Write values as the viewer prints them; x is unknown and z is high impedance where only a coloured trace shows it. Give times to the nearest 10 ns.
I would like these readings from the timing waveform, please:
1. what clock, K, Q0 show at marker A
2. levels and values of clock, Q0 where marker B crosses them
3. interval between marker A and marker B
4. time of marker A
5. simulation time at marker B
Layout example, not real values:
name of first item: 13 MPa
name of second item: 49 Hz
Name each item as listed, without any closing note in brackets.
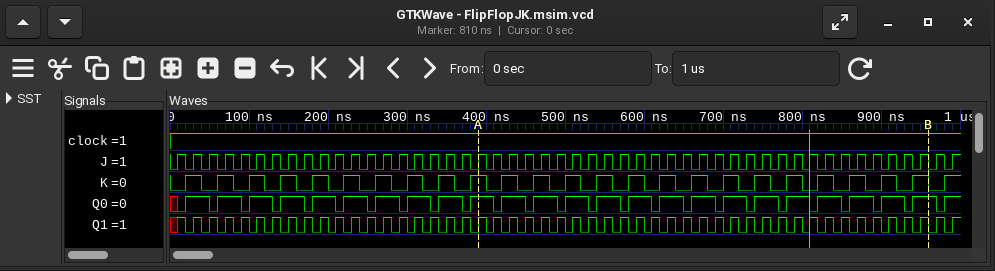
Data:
what clock, K, Q0 show at marker A: clock=1, K=1, Q0=1
levels and values of clock, Q0 where marker B crosses them: clock=1, Q0=1
interval between marker A and marker B: 570 ns
time of marker A: 390 ns
simulation time at marker B: 960 ns
